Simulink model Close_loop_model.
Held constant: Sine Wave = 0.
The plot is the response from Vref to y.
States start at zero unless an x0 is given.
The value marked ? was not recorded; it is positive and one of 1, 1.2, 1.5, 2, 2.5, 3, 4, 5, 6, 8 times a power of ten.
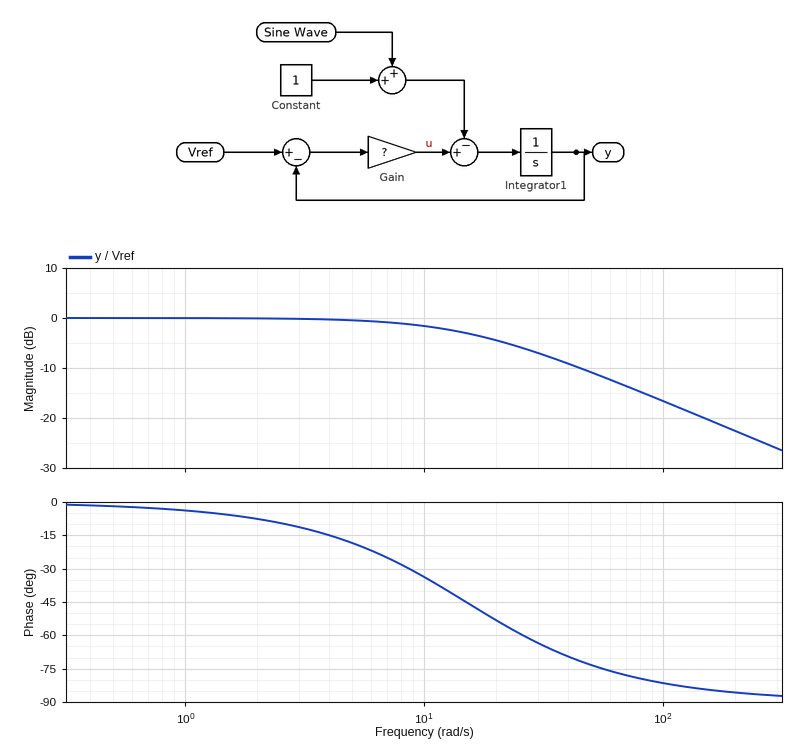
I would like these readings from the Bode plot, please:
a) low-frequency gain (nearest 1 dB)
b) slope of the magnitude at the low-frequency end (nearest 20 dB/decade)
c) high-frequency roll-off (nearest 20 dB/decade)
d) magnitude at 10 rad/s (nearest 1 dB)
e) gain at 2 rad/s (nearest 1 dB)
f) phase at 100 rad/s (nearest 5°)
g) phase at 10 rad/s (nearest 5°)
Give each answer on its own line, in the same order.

0 dB
0 dB/decade
-20 dB/decade
-2 dB
0 dB
-80°
-35°
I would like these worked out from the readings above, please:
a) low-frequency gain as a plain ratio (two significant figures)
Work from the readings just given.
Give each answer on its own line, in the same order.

1.0
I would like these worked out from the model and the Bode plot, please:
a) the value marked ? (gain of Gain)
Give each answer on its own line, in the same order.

15
